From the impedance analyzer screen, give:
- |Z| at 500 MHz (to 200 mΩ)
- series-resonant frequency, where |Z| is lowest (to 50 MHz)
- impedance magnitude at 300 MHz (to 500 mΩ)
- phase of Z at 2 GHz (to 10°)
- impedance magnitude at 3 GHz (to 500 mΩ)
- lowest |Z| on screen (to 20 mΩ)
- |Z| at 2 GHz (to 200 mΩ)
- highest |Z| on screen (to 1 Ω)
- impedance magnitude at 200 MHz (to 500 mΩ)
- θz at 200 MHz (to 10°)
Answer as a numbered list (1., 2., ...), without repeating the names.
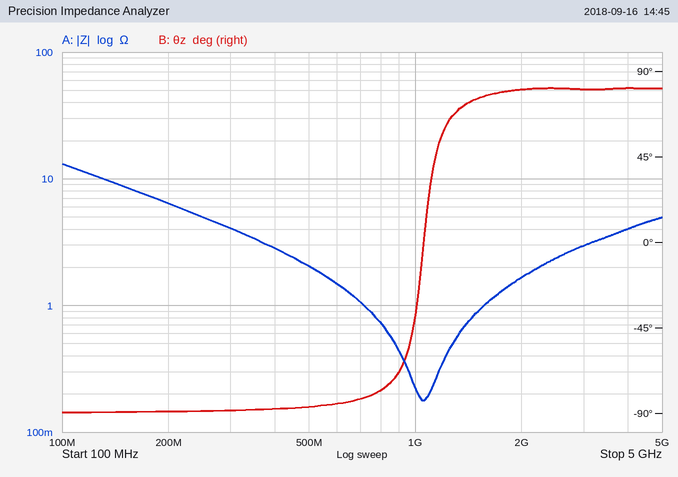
1. 2.0 Ω
2. 1.05 GHz
3. 4.0 Ω
4. 80°
5. 3.0 Ω
6. 180 mΩ
7. 1.6 Ω
8. 13 Ω
9. 6.5 Ω
10. -90°
